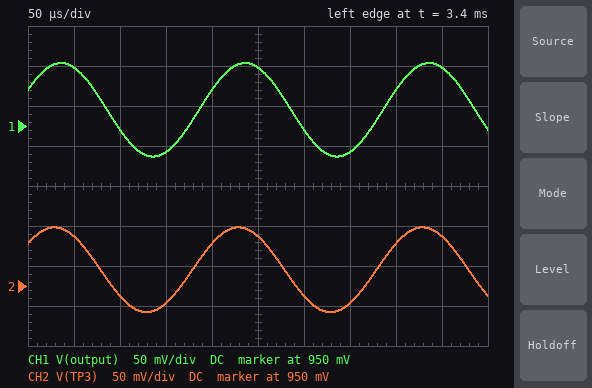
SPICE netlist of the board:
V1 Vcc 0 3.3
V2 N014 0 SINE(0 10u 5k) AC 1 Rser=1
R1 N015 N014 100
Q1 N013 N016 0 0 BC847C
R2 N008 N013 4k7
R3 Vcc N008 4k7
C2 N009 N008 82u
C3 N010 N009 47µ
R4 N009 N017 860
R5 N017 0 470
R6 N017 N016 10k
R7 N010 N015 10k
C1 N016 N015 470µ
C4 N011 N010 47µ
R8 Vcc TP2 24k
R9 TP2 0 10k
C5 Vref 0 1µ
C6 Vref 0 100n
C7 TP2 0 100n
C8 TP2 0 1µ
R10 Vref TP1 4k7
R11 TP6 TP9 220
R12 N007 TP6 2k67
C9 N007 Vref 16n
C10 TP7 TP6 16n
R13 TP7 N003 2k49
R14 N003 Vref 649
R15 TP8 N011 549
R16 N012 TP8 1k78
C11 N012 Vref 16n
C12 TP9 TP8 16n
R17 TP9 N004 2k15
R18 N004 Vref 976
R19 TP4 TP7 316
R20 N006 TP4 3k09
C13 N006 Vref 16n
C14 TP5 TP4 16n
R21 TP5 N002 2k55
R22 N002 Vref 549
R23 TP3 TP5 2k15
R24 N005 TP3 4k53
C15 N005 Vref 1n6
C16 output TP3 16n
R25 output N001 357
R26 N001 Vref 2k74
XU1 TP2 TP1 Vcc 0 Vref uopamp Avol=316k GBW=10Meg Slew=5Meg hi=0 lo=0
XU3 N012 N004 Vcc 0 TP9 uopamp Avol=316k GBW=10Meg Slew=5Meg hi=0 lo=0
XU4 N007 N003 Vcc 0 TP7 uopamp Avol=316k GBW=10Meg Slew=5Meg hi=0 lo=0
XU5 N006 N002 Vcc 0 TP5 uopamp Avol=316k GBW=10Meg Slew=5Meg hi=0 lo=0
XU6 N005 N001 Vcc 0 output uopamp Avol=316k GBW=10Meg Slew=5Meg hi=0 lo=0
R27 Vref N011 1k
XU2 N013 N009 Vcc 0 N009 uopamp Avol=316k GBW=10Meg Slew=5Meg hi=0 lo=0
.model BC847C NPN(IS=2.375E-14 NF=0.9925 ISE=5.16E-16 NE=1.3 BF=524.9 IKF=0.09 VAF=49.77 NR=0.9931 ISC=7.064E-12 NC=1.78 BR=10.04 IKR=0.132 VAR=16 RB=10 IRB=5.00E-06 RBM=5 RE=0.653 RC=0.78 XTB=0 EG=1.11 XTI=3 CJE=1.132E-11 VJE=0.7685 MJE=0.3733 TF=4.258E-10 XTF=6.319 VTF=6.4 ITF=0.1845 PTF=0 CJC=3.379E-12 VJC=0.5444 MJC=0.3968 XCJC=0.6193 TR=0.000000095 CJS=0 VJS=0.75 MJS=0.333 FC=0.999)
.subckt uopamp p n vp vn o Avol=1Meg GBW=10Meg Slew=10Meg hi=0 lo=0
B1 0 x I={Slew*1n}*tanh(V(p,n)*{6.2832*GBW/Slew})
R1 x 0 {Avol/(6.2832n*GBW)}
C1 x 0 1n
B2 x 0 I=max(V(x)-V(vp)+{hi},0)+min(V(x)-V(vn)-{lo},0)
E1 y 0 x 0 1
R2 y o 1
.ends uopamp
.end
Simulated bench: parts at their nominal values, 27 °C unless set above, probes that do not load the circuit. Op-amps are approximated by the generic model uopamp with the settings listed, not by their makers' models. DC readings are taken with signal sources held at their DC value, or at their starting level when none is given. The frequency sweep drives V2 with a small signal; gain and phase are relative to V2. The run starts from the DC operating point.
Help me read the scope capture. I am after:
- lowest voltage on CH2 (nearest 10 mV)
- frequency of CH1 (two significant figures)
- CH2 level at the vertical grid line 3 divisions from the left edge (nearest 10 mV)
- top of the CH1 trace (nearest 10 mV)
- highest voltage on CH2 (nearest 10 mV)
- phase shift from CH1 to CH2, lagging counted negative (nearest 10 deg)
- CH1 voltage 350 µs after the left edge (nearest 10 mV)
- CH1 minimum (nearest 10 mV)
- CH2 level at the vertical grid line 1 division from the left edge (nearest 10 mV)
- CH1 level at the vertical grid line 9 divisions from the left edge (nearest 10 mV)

920 mV
5.0 kHz
930 mV
1.03 V
1.02 V
10 deg
920 mV
910 mV
1.01 V
1.02 V
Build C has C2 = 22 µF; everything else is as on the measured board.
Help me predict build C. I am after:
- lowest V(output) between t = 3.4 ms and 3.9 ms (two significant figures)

910 mV
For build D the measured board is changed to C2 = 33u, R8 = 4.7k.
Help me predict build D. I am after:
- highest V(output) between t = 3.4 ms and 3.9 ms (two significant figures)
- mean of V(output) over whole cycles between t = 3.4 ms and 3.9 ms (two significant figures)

2.3 V
2.2 V
